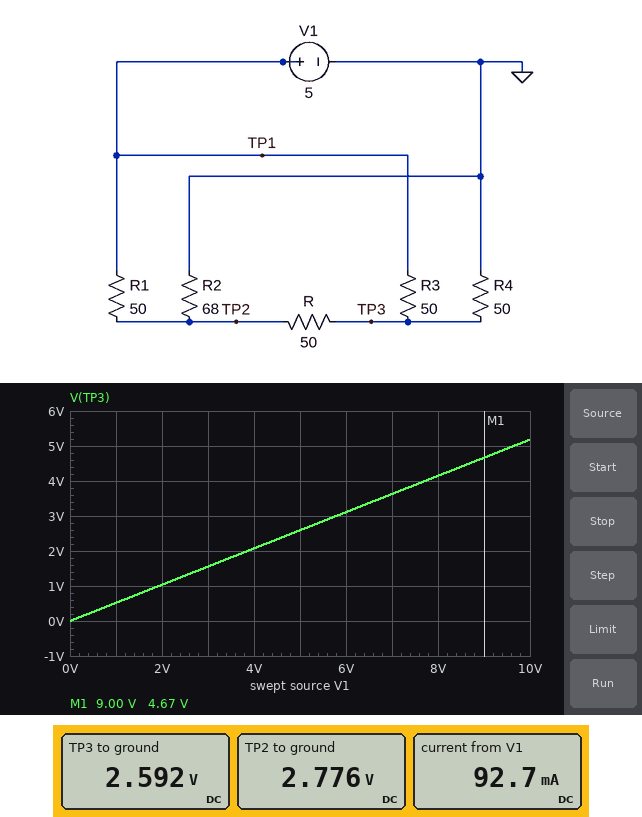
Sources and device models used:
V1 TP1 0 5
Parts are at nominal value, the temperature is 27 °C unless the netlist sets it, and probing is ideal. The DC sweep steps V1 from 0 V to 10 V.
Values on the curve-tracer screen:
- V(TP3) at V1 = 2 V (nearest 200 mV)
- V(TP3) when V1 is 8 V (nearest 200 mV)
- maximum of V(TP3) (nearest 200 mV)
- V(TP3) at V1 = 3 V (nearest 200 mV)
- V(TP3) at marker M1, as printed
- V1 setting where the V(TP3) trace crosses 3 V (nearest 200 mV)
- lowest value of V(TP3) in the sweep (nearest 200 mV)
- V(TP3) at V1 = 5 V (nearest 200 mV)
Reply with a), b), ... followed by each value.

a) 1.0 V
b) 4.2 V
c) 5.2 V
d) 1.6 V
e) 4.67 V
f) 5.8 V
g) 0 V
h) 2.6 V
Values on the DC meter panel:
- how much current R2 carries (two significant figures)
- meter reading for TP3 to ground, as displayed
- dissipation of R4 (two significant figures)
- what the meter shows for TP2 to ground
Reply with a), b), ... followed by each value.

a) 41 mA
b) 2.592 V
c) 130 mW
d) 2.776 V
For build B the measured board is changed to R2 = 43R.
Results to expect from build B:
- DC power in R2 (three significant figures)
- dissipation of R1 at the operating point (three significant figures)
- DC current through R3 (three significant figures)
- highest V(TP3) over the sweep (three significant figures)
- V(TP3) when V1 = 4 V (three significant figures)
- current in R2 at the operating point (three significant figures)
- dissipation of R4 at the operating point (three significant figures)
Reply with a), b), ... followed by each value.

a) 129 mW
b) 140 mW
c) 51.0 mA
d) 4.90 V
e) 1.96 V
f) 54.8 mA
g) 120 mW
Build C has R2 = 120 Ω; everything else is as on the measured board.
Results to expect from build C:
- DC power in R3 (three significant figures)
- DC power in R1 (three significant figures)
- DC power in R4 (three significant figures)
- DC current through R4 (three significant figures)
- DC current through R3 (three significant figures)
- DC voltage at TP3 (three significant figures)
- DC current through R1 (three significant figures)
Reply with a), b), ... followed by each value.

a) 103 mW
b) 64.8 mW
c) 149 mW
d) 54.7 mA
e) 45.3 mA
f) 2.73 V
g) 36.0 mA
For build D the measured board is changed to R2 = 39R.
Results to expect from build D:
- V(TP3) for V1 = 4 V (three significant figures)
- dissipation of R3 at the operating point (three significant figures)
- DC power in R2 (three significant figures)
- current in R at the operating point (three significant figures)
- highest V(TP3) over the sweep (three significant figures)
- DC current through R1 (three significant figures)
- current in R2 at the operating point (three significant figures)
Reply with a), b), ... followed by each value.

a) 1.94 V
b) 133 mW
c) 131 mW
d) 3.19 mA
e) 4.84 V
f) 54.8 mA
g) 58.0 mA
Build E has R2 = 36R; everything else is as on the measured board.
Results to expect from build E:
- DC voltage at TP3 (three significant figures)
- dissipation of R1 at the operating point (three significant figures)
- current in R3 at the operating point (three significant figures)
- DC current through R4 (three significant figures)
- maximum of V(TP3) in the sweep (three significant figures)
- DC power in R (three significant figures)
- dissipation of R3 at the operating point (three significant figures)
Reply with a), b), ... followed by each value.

a) 2.39 V
b) 159 mW
c) 52.1 mA
d) 47.9 mA
e) 4.79 V
f) 900 µW
g) 136 mW
